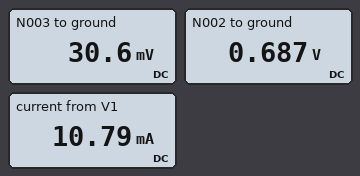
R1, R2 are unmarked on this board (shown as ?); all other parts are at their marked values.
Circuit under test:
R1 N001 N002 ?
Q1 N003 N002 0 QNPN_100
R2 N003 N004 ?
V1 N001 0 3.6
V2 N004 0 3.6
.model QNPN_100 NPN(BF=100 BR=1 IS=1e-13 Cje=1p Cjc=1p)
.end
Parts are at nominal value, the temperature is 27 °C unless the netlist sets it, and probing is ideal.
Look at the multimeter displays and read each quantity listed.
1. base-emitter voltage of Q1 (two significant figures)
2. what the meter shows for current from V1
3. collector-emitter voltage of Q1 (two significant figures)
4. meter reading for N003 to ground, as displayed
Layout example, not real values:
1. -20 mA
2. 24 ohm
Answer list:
1. 690 mV
2. 10.79 mA
3. 31 mV
4. 30.6 mV
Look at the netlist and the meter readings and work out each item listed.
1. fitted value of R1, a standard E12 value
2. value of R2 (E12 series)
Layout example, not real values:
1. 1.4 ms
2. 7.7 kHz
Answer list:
1. 270 Ω
2. 270 Ω
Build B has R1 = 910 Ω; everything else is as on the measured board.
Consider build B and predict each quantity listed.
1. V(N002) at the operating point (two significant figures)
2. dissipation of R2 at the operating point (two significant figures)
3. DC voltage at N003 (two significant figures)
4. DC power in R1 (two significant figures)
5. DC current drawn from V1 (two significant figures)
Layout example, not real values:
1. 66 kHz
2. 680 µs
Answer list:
1. 670 mV
2. 47 mW
3. 48 mV
4. 9.4 mW
5. 3.2 mA
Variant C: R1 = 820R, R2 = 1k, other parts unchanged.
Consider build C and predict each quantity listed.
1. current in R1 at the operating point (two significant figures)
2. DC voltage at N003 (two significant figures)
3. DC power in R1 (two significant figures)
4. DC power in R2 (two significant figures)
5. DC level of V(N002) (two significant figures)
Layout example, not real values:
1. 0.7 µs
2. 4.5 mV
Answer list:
1. 3.6 mA
2. 29 mV
3. 11 mW
4. 13 mW
5. 660 mV
